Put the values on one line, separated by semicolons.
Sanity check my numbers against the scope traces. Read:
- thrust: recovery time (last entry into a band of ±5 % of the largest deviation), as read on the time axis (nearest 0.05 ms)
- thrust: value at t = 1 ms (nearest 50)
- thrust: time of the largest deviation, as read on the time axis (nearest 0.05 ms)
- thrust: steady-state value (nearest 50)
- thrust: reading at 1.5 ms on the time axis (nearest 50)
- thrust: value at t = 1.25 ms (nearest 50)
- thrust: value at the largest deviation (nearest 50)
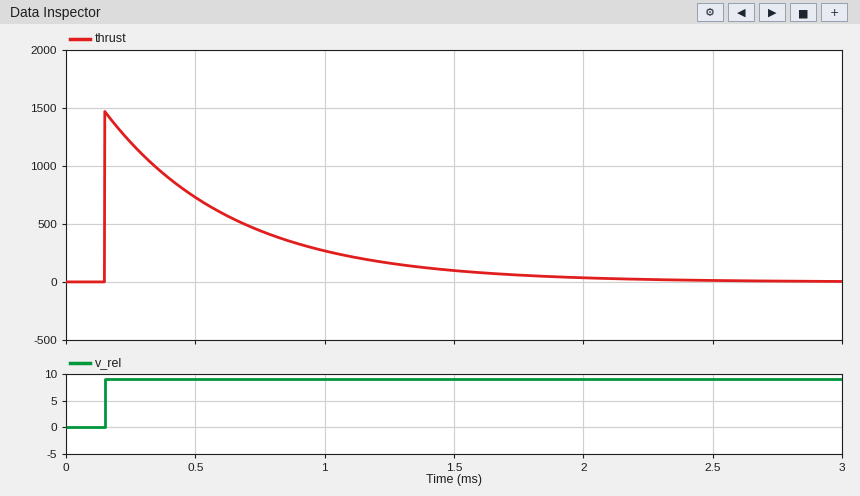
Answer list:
1.65 ms; 250; 0.15 ms; 0; 100; 150; 1450
